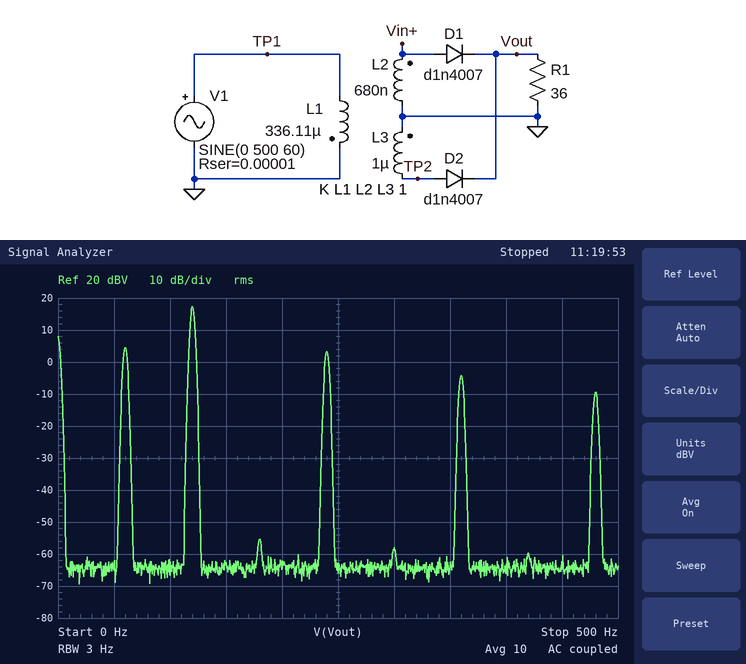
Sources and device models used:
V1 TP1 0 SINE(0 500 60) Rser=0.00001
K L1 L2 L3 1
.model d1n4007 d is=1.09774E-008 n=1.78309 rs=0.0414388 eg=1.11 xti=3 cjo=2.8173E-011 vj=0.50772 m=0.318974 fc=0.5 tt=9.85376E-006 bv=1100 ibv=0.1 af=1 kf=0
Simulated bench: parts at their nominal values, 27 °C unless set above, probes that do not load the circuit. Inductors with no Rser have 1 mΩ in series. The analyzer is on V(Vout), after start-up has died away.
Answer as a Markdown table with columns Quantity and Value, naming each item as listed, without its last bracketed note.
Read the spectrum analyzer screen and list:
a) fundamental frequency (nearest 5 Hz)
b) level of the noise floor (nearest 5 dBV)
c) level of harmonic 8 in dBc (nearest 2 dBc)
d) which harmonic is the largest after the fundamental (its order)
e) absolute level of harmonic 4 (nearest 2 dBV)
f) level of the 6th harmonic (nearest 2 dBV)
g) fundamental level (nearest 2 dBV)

| Quantity | Value |
|---|---|
| fundamental frequency | 60 Hz |
| level of the noise floor | -65 dBV |
| level of harmonic 8 in dBc | -14 dBc |
| which harmonic is the largest after the fundamental | 2 |
| absolute level of harmonic 4 | 4 dBV |
| level of the 6th harmonic | -4 dBV |
| fundamental level | 4 dBV |
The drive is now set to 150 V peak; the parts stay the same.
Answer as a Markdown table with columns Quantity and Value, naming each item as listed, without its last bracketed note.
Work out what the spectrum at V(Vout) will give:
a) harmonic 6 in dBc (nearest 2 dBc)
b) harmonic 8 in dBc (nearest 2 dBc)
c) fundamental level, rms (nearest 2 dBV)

| Quantity | Value |
|---|---|
| harmonic 6 in dBc | -10 dBc |
| harmonic 8 in dBc | -16 dBc |
| fundamental level, rms | -6 dBV |
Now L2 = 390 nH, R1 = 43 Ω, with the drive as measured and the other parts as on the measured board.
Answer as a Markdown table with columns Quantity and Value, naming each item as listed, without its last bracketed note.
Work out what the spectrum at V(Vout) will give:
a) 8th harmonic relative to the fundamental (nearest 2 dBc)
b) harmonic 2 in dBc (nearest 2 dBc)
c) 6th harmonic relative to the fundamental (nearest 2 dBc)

| Quantity | Value |
|---|---|
| 8th harmonic relative to the fundamental | -22 dBc |
| harmonic 2 in dBc | 6 dBc |
| 6th harmonic relative to the fundamental | -16 dBc |
